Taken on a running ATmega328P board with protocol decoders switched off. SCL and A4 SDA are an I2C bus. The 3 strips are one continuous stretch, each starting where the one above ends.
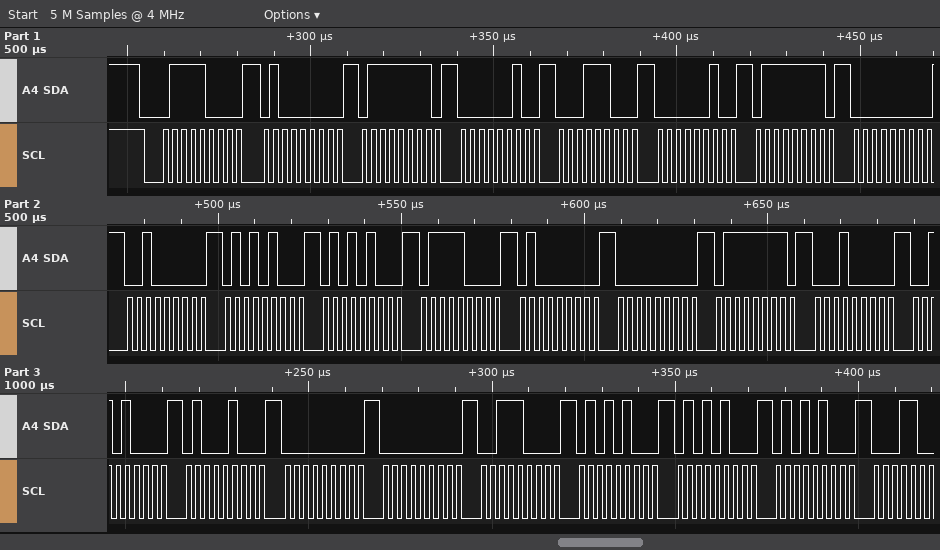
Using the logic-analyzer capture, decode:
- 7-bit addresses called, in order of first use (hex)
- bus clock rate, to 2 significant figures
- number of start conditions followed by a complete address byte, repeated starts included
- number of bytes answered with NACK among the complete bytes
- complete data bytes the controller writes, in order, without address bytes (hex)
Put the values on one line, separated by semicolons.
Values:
0x3C; 400 kHz; 1; 0; 40 7F 02 1C 02 7F 00 20 54 54 78 40 00 7F 10 28 44 00 00 38 54 54 54
